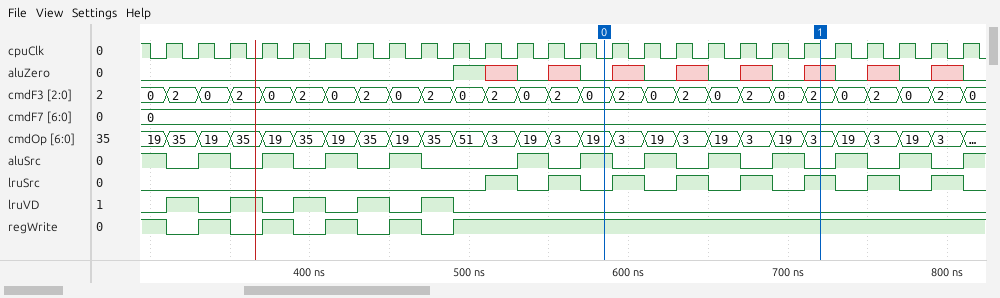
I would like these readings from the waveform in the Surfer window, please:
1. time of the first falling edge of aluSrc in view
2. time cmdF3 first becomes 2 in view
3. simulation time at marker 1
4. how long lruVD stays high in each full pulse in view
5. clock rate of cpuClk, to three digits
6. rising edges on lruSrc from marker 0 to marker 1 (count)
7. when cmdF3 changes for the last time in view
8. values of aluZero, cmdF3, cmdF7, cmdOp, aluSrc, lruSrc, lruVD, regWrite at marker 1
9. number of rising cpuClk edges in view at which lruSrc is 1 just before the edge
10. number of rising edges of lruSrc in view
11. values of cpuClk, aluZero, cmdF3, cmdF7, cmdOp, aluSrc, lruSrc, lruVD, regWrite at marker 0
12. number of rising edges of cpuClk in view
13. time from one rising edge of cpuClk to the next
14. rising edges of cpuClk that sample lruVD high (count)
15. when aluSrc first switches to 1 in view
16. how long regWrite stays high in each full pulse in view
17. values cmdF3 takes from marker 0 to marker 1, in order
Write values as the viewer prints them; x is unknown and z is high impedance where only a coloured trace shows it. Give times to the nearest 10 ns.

310 ns
310 ns
720 ns
20 ns, 20 ns, 20 ns, 20 ns, 20 ns
50.0 MHz
4
810 ns
aluZero=x, cmdF3=2, cmdF7=0, cmdOp=3, aluSrc=0, lruSrc=1, lruVD=0, regWrite=1
8
8
cpuClk=0, aluZero=0, cmdF3=0, cmdF7=0, cmdOp=19, aluSrc=1, lruSrc=0, lruVD=0, regWrite=1
26
20 ns
5
330 ns
20 ns, 20 ns, 20 ns, 20 ns
0, 2, 0, 2, 0, 2, 0, 2
